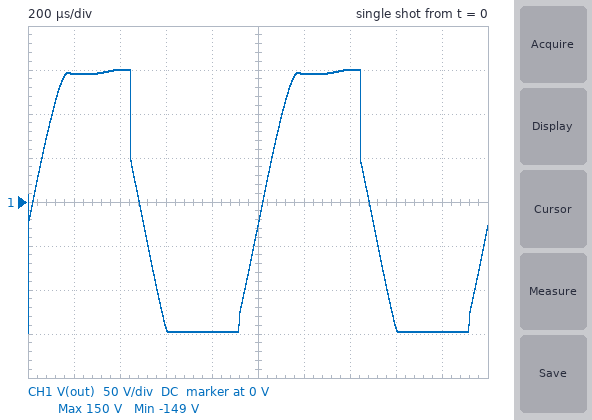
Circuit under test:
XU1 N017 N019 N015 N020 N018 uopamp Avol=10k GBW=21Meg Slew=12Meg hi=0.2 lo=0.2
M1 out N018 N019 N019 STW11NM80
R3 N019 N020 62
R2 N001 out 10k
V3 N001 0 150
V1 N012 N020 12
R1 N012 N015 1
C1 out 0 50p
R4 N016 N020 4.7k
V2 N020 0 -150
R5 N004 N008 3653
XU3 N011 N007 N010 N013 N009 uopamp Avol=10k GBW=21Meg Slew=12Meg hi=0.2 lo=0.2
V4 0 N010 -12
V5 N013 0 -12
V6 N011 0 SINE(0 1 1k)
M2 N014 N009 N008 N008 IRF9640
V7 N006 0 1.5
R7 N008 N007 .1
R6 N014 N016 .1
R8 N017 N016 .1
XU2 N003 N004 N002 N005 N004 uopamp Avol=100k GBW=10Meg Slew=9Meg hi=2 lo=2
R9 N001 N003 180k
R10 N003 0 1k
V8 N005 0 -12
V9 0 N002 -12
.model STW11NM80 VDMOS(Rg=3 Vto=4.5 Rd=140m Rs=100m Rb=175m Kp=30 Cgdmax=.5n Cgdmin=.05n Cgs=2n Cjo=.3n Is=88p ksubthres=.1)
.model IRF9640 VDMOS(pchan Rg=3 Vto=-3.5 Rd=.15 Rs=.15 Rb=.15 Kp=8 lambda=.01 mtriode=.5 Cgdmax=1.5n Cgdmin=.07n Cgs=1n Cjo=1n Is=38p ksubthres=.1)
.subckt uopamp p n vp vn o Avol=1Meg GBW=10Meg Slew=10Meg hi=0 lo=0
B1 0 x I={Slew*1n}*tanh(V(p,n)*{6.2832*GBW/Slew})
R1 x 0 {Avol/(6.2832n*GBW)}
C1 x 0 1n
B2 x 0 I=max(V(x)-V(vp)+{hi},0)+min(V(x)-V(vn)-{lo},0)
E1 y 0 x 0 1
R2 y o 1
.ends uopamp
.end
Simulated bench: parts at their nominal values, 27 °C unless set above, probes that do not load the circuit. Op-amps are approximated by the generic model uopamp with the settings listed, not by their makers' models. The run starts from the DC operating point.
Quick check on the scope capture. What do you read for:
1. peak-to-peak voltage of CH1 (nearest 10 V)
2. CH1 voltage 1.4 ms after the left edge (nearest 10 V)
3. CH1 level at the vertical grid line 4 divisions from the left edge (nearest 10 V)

300 V
150 V
-150 V
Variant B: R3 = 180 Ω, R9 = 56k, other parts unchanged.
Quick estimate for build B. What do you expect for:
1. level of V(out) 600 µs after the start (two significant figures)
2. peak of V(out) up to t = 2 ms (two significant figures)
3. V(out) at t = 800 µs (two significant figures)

-80 V
33 V
-110 V
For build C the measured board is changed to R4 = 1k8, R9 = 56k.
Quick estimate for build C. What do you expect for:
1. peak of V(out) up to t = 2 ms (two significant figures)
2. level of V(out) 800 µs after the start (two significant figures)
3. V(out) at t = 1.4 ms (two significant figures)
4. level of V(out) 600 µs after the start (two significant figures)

18 V
-140 V
-14 V
-110 V
